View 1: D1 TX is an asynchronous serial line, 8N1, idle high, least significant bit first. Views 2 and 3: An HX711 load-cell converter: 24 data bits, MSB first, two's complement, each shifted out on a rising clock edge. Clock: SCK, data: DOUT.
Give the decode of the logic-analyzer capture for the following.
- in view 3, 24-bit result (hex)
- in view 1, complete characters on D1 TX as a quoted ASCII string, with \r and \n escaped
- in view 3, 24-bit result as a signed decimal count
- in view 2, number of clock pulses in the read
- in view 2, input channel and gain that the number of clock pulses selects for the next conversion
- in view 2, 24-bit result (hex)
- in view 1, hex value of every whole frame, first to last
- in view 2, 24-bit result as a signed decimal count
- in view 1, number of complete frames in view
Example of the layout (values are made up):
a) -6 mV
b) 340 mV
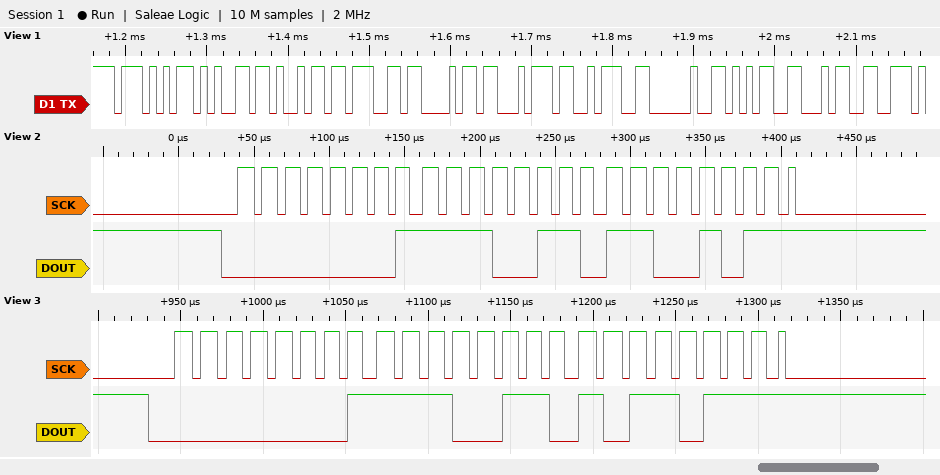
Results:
a) 0x01E6B7
b) "Weight: 54"
c) 124599
d) 25
e) channel A, gain 128
f) 0x01E6CB
g) 57 65 69 67 68 74 3A 20 35 34
h) 124619
i) 10
